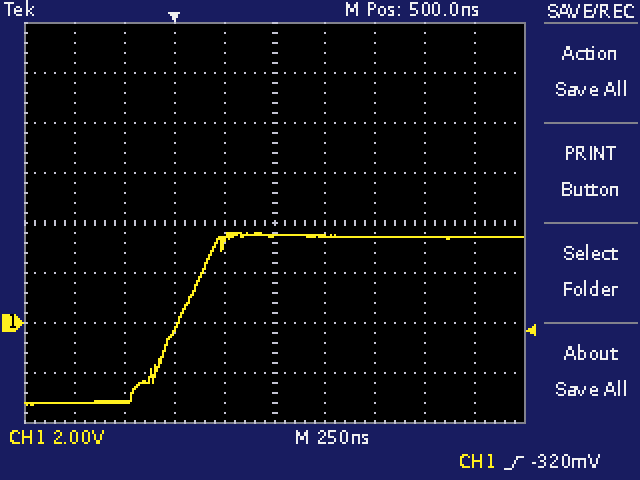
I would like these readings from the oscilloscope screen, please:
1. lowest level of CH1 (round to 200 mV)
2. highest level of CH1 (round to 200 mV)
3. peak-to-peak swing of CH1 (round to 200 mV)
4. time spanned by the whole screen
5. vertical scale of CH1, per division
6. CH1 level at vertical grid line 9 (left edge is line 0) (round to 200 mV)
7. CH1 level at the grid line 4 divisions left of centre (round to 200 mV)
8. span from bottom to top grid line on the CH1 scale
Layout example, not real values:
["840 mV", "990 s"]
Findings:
["-3.2 V", "3.6 V", "6.8 V", "2.5 µs", "2 V", "3.4 V", "-3.2 V", "16 V"]
